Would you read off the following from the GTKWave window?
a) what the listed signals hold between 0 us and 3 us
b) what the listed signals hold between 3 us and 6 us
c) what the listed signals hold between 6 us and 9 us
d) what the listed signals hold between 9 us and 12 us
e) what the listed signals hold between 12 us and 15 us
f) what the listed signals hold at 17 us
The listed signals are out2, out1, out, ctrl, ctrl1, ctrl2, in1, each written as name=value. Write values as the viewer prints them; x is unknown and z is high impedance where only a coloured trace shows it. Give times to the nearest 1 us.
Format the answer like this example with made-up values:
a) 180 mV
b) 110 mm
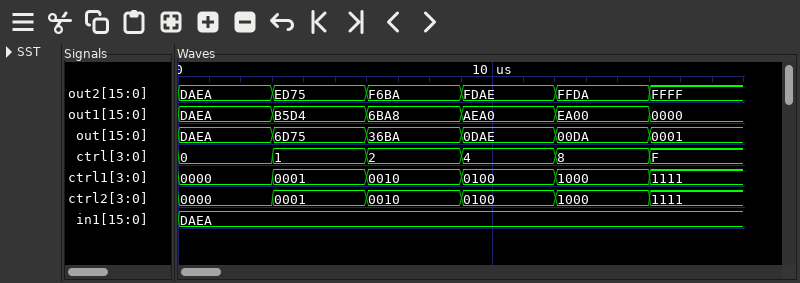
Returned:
a) out2=DAEA, out1=DAEA, out=DAEA, ctrl=0, ctrl1=0000, ctrl2=0000, in1=DAEA
b) out2=ED75, out1=B5D4, out=6D75, ctrl=1, ctrl1=0001, ctrl2=0001, in1=DAEA
c) out2=F6BA, out1=6BA8, out=36BA, ctrl=2, ctrl1=0010, ctrl2=0010, in1=DAEA
d) out2=FDAE, out1=AEA0, out=0DAE, ctrl=4, ctrl1=0100, ctrl2=0100, in1=DAEA
e) out2=FFDA, out1=EA00, out=00DA, ctrl=8, ctrl1=1000, ctrl2=1000, in1=DAEA
f) out2=FFFF, out1=0000, out=0001, ctrl=F, ctrl1=1111, ctrl2=1111, in1=DAEA
